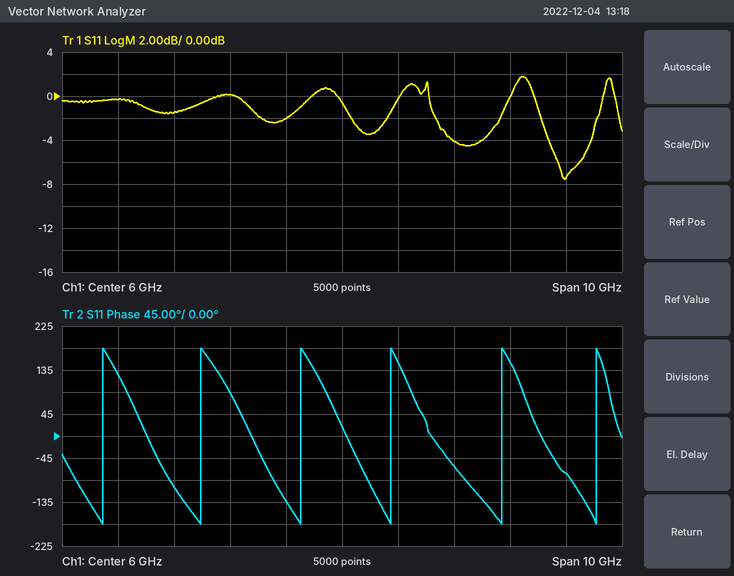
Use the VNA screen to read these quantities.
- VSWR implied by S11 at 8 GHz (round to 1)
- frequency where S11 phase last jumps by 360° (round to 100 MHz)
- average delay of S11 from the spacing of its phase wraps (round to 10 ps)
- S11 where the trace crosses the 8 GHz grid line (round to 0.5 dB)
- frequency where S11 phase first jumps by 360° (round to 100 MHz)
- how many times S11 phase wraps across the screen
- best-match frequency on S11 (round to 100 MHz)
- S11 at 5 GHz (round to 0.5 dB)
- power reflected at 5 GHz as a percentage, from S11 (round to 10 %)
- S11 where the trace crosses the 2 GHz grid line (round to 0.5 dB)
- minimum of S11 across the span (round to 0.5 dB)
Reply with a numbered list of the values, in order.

1. 4
2. 10.5 GHz
3. 570 ps
4. -4.0 dB
5. 1.7 GHz
6. 6
7. 10.0 GHz
8. -2.0 dB
9. 60 %
10. -0.5 dB
11. -7.5 dB
